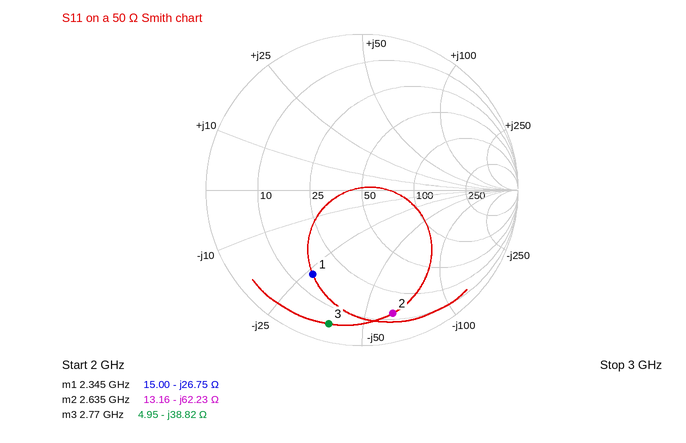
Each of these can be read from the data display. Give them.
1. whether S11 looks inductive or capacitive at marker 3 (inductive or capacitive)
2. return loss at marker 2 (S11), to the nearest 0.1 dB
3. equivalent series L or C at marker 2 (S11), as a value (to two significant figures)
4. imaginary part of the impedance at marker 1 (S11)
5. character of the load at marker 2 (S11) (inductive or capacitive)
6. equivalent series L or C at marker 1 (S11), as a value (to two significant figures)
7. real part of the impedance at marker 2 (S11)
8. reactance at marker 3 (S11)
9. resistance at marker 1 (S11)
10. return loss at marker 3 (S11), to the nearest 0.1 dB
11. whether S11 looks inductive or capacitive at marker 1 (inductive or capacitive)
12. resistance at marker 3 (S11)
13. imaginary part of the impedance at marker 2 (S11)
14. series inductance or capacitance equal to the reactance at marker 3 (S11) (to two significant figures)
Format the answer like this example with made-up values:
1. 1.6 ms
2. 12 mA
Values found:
1. capacitive
2. 1.8 dB
3. 970 fF
4. -26.75 Ω
5. capacitive
6. 2.5 pF
7. 13.16 Ω
8. -38.82 Ω
9. 15.00 Ω
10. 1.1 dB
11. capacitive
12. 4.95 Ω
13. -62.23 Ω
14. 1.5 pF
